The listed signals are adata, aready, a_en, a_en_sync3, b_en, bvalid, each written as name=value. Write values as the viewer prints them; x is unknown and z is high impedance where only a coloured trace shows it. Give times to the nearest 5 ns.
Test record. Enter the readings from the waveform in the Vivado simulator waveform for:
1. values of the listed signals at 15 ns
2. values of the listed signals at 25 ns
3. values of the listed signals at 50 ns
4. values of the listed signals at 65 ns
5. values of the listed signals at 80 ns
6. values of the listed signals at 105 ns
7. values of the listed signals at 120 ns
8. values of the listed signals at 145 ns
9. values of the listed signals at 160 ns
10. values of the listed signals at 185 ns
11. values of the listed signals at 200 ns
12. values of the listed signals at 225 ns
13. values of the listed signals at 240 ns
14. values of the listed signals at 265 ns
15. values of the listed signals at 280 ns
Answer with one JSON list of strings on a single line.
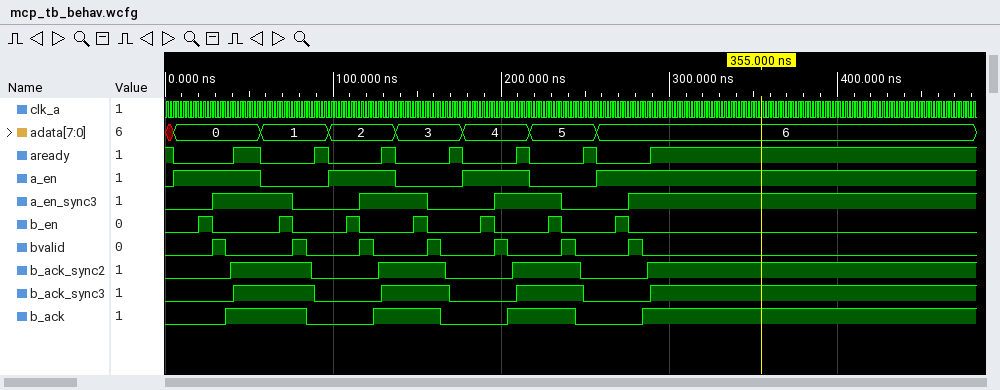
["adata=0, aready=0, a_en=1, a_en_sync3=0, b_en=0, bvalid=0", "adata=0, aready=0, a_en=1, a_en_sync3=0, b_en=1, bvalid=0", "adata=0, aready=1, a_en=1, a_en_sync3=1, b_en=0, bvalid=0", "adata=1, aready=0, a_en=0, a_en_sync3=1, b_en=0, bvalid=0", "adata=1, aready=0, a_en=0, a_en_sync3=0, b_en=0, bvalid=1", "adata=2, aready=0, a_en=1, a_en_sync3=0, b_en=0, bvalid=0", "adata=2, aready=0, a_en=1, a_en_sync3=1, b_en=0, bvalid=1", "adata=3, aready=0, a_en=0, a_en_sync3=1, b_en=0, bvalid=0", "adata=3, aready=0, a_en=0, a_en_sync3=0, b_en=0, bvalid=1", "adata=4, aready=0, a_en=1, a_en_sync3=0, b_en=0, bvalid=0", "adata=4, aready=0, a_en=1, a_en_sync3=1, b_en=0, bvalid=1", "adata=5, aready=0, a_en=0, a_en_sync3=1, b_en=0, bvalid=0", "adata=5, aready=0, a_en=0, a_en_sync3=0, b_en=0, bvalid=1", "adata=6, aready=0, a_en=1, a_en_sync3=0, b_en=0, bvalid=0", "adata=6, aready=0, a_en=1, a_en_sync3=1, b_en=0, bvalid=1"]
